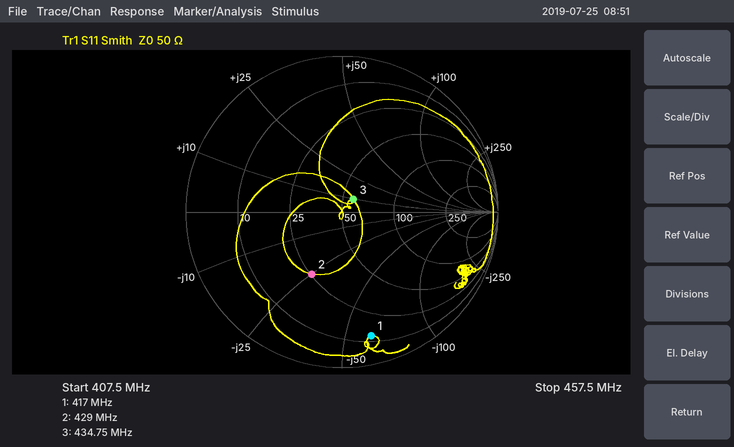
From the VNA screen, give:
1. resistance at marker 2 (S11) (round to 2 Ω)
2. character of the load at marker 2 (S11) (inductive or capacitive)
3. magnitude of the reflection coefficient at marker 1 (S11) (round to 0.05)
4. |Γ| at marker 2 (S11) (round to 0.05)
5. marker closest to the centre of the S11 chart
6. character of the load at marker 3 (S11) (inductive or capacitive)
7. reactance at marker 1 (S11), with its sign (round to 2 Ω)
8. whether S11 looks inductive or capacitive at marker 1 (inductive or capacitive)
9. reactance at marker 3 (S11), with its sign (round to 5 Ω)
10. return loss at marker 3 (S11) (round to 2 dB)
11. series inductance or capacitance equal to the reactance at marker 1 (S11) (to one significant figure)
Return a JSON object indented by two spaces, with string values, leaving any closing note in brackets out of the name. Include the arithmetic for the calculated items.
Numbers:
{
  "resistance at marker 2 (S11)": "26 Ω",
  "character of the load at marker 2 (S11)": "capacitive",
  "magnitude of the reflection coefficient at marker 1 (S11)": "0.80",
  "|Γ| at marker 2 (S11)": "0.45",
  "marker closest to the centre of the S11 chart": "marker 3",
  "character of the load at marker 3 (S11)": "inductive",
  "reactance at marker 1 (S11), with its sign": "-62 Ω",
  "whether S11 looks inductive or capacitive at marker 1": "capacitive",
  "reactance at marker 3 (S11), with its sign": "+10 Ω",
  "return loss at marker 3 (S11)": "20 dB",
  "series inductance or capacitance equal to the reactance at marker 1 (S11)": "C = 1/(2π × 417 MHz × 62 Ω) ≈ 6 pF"
}
